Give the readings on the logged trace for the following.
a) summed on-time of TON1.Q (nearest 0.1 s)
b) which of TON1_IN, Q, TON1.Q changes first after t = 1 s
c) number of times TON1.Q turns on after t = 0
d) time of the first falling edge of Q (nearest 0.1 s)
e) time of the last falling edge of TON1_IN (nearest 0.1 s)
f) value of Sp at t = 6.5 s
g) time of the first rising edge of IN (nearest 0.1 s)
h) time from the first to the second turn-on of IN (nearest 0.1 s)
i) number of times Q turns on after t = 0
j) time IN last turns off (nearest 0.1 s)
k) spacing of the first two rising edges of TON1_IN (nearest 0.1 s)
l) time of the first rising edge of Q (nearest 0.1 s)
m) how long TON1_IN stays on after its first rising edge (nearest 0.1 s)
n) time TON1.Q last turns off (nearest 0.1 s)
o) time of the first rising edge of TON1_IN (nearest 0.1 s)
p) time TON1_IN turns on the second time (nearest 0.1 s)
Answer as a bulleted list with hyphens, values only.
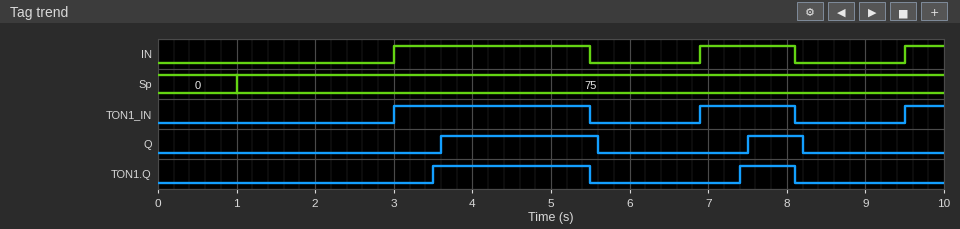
- 2.7 s
- TON1_IN
- 2
- 5.6 s
- 8.1 s
- 75
- 3.0 s
- 3.9 s
- 2
- 8.1 s
- 3.9 s
- 3.6 s
- 2.5 s
- 8.1 s
- 3.0 s
- 6.9 s
